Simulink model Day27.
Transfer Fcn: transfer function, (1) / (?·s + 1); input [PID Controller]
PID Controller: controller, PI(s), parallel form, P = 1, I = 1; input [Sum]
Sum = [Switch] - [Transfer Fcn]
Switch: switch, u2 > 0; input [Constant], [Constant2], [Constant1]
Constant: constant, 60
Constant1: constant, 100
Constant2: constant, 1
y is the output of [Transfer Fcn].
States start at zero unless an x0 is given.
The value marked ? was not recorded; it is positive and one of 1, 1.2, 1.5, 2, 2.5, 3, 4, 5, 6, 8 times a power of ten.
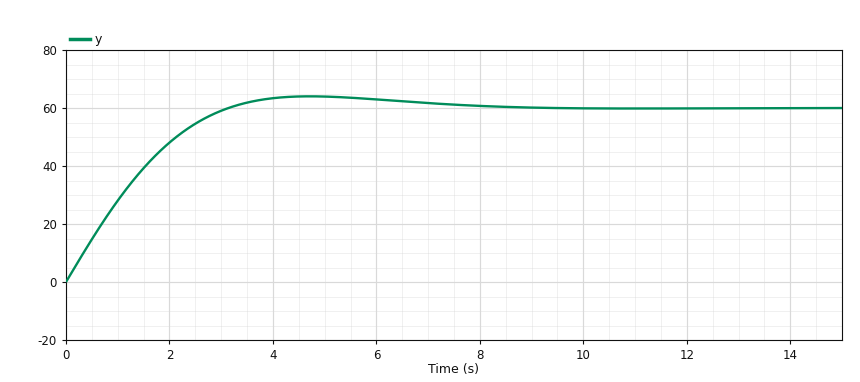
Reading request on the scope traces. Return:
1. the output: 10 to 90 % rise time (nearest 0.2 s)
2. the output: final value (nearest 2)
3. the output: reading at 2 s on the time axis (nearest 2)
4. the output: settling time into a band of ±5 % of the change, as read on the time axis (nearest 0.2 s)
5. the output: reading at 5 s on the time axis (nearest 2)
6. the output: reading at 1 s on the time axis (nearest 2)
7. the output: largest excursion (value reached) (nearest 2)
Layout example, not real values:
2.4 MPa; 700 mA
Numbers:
2.2 s; 60; 48; 6.0 s; 64; 28; 64
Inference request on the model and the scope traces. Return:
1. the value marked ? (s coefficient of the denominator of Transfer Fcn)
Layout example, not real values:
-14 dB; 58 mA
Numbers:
2
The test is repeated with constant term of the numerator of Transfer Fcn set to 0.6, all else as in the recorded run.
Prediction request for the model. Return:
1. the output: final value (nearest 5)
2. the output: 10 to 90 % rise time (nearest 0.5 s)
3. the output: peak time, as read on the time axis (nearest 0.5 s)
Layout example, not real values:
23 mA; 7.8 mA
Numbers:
60; 3.5 s; 7.0 s
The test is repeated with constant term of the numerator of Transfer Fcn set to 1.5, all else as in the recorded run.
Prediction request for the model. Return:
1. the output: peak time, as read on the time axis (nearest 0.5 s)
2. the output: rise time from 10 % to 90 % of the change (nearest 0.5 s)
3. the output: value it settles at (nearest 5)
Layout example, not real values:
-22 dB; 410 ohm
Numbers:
3.5 s; 1.5 s; 60
